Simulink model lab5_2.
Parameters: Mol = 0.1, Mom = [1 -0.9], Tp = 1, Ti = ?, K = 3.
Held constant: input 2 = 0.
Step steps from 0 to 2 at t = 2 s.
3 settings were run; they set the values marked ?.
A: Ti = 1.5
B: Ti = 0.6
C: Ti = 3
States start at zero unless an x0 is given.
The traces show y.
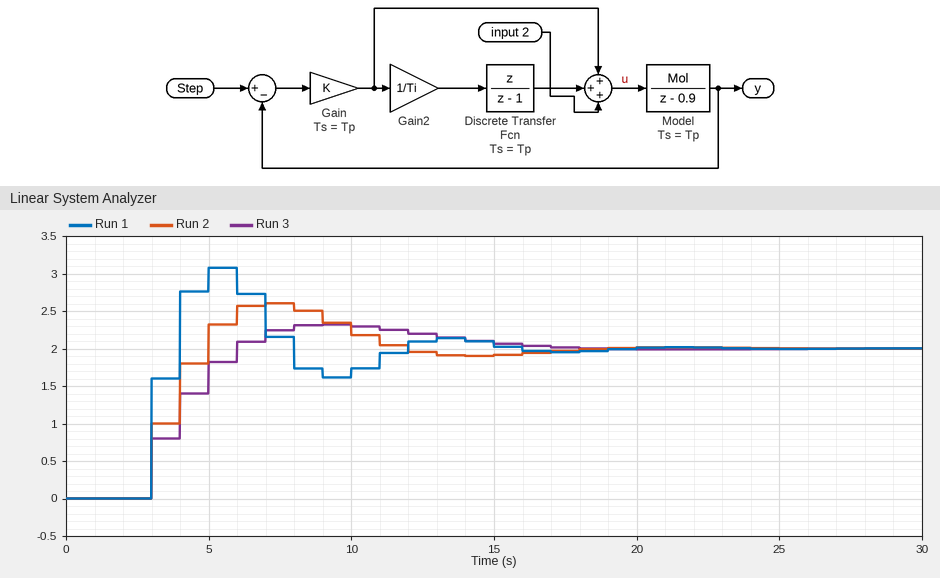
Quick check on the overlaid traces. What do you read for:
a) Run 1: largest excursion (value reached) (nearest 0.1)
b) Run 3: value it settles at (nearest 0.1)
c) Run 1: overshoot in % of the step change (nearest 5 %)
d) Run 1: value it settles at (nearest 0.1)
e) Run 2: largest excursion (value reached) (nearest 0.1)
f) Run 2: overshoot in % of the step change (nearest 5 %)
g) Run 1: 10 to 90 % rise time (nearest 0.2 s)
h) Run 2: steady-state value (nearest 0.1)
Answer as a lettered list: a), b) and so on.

a) 3.1
b) 2.0
c) 55 %
d) 2.0
e) 2.6
f) 30 %
g) 1.0 s
h) 2.0
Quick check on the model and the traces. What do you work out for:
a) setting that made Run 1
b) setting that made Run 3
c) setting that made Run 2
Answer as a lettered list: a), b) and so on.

a) B
b) C
c) A
